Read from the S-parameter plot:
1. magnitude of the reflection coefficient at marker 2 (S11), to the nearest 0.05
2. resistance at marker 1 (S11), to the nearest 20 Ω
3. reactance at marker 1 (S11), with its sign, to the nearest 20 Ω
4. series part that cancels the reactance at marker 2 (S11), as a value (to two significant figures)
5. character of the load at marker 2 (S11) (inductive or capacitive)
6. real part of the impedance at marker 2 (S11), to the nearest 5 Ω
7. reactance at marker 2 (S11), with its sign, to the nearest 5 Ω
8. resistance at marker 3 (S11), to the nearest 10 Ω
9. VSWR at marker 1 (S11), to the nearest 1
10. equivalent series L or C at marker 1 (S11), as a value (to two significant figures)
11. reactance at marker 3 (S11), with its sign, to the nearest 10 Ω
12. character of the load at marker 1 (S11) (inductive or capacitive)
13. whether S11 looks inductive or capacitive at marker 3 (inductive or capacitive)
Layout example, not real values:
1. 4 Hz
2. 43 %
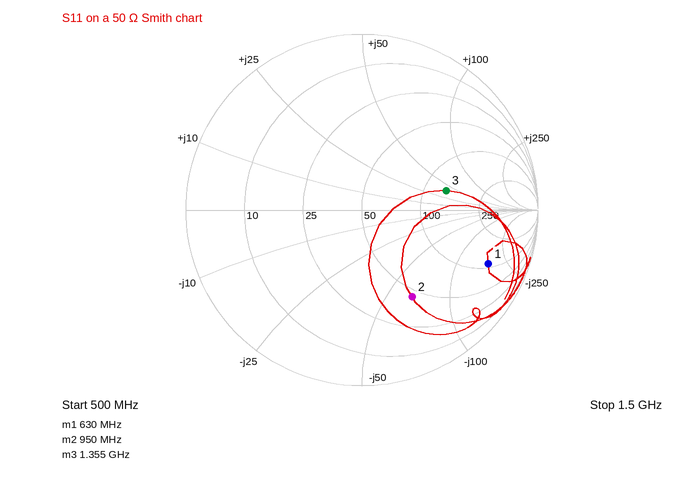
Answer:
1. 0.55
2. 120 Ω
3. -180 Ω
4. 11 nH
5. capacitive
6. 45 Ω
7. -65 Ω
8. 130 Ω
9. 8
10. 1.4 pF
11. +40 Ω
12. capacitive
13. inductive
